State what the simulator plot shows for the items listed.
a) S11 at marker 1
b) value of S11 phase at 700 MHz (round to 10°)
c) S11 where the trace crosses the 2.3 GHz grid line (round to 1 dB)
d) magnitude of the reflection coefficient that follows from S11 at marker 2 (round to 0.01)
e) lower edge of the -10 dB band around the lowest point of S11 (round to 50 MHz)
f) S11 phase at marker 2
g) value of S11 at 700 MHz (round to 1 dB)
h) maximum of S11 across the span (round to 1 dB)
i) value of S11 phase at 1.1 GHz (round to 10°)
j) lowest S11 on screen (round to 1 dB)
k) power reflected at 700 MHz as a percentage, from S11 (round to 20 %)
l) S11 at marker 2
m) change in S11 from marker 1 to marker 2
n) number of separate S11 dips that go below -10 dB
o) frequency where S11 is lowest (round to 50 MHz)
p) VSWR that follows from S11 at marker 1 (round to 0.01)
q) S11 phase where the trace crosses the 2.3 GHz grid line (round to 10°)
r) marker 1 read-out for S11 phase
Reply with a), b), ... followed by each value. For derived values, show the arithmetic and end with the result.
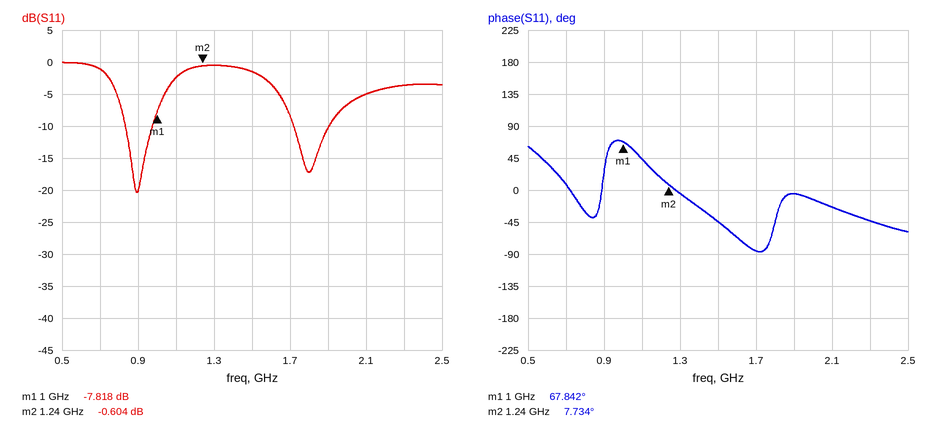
a) -7.818 dB
b) 10°
c) -4 dB
d) 10^(-0.604/20) ≈ 0.93
e) 850 MHz
f) 7.734°
g) -1 dB
h) 0 dB
i) 40°
j) -20 dB
k) 10^(-1/10) ≈ 79.4 %, so 80 % to the nearest 20 %
l) -0.604 dB
m) -0.604 − (-7.818) = 7.214 dB
n) 2
o) 900 MHz
p) (1 + 0.4065)/(1 − 0.4065) ≈ 2.37
q) -40°
r) 67.842°
